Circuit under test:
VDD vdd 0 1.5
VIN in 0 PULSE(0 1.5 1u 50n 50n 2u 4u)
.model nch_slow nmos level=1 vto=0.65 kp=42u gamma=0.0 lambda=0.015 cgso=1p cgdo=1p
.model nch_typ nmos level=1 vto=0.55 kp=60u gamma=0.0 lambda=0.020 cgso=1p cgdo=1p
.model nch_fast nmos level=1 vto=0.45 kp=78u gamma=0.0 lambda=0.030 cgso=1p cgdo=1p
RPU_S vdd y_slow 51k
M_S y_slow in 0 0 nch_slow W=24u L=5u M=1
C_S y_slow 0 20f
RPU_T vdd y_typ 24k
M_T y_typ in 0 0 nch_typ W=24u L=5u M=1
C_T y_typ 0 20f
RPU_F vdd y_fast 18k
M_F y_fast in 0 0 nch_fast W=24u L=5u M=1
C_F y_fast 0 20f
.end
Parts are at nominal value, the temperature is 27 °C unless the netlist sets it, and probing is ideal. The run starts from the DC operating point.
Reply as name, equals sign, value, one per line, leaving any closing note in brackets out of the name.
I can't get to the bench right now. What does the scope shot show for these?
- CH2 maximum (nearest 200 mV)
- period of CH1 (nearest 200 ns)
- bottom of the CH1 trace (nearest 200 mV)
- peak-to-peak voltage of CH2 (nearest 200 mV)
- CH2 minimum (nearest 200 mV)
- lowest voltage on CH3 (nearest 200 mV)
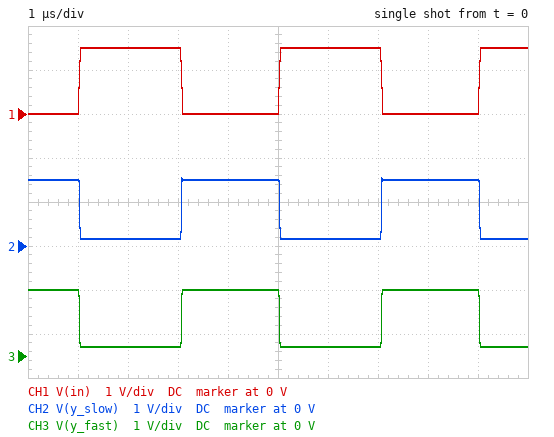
CH2 maximum = 1.6 V
period of CH1 = 4.0 µs
bottom of the CH1 trace = 0 V
peak-to-peak voltage of CH2 = 1.4 V
CH2 minimum = 200 mV
lowest voltage on CH3 = 200 mV
